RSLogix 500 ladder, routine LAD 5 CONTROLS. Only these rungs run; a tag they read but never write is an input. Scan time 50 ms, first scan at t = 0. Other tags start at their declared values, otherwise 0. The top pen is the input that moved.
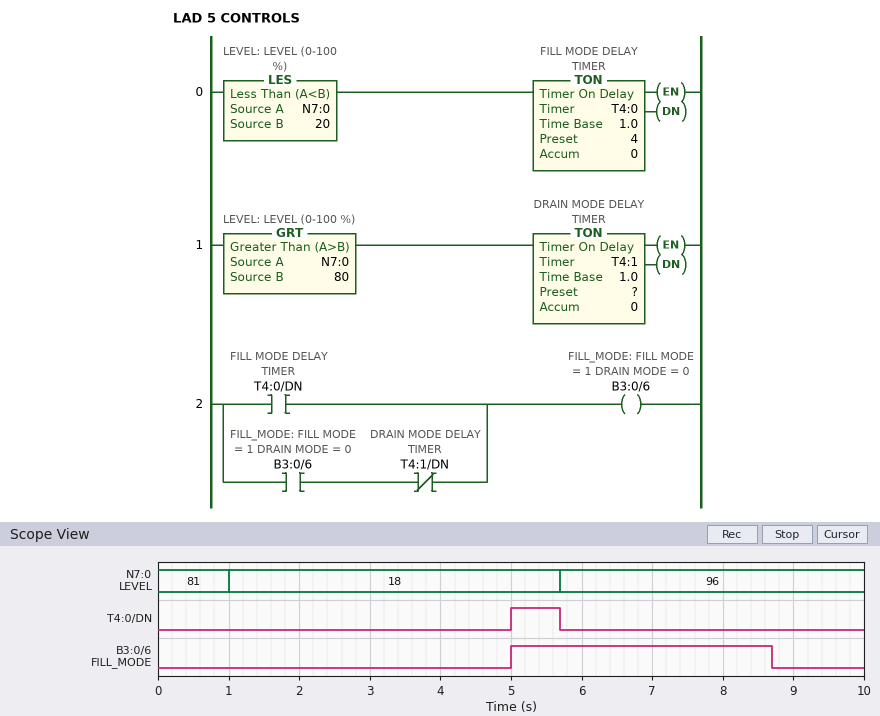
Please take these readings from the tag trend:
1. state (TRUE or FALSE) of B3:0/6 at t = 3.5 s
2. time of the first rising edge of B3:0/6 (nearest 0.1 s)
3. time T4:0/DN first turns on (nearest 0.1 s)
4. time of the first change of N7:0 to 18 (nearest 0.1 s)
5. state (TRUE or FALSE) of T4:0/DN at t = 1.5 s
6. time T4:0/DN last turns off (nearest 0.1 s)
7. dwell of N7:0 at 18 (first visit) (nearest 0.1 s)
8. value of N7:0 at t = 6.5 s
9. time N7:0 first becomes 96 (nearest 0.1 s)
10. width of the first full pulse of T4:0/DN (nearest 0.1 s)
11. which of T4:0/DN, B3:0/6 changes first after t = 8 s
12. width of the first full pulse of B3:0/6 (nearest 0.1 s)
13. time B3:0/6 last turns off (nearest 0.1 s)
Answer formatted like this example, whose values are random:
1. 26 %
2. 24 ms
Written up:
1. FALSE
2. 5.0 s
3. 5.0 s
4. 1.0 s
5. FALSE
6. 5.7 s
7. 4.7 s
8. 96
9. 5.7 s
10. 0.7 s
11. B3:0/6
12. 3.7 s
13. 8.7 s
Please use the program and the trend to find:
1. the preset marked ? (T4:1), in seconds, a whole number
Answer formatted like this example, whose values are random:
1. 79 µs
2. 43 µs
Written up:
1. 3 s
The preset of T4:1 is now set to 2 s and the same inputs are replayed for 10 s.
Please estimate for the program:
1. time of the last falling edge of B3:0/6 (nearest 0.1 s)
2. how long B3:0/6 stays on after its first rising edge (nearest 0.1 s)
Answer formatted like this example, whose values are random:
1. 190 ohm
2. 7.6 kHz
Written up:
1. 7.7 s
2. 2.7 s
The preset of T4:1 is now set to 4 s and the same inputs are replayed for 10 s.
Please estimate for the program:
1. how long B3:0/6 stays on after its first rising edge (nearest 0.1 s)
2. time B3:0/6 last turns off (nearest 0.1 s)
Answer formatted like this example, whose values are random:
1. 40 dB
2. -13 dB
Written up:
1. 4.7 s
2. 9.7 s
